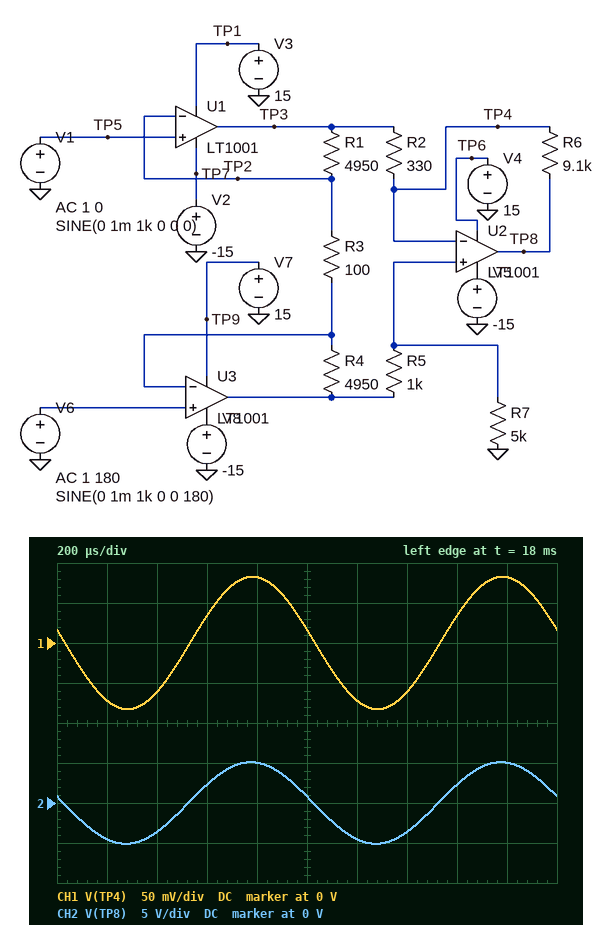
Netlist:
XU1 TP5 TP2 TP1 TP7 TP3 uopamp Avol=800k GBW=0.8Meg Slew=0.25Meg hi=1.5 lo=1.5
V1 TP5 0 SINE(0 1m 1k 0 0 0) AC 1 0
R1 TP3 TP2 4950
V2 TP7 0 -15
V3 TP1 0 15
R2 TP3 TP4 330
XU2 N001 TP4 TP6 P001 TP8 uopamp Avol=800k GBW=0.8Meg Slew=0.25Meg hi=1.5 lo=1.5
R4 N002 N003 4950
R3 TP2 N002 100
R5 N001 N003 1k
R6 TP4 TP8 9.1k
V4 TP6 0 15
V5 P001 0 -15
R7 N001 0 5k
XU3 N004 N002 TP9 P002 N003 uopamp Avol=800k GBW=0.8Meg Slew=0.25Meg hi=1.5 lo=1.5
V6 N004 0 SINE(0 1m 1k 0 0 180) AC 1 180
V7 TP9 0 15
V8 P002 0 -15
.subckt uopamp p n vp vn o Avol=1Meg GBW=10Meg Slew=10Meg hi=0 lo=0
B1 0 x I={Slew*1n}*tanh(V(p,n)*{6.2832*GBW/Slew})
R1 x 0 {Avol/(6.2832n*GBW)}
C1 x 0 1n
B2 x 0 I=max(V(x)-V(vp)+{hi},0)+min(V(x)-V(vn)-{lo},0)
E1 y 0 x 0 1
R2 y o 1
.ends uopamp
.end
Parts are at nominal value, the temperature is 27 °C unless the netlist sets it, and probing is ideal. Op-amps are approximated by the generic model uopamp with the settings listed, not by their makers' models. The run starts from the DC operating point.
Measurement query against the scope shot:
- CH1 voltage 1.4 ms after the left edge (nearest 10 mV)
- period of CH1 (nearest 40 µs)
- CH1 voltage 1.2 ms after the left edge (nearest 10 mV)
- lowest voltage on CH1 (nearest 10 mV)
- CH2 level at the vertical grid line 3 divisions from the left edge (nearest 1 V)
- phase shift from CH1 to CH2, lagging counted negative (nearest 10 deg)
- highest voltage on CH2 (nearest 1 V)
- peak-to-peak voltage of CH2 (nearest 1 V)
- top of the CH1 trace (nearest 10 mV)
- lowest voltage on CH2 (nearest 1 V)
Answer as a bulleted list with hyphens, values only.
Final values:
- -60 mV
- 1.00 ms
- -70 mV
- -80 mV
- 2 V
- 0 deg
- 5 V
- 10 V
- 80 mV
- -5 V
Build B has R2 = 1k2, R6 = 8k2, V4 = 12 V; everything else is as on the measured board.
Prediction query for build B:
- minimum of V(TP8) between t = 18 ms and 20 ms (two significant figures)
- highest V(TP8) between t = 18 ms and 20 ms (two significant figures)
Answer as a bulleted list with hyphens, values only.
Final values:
- -1.3 V
- 1.3 V
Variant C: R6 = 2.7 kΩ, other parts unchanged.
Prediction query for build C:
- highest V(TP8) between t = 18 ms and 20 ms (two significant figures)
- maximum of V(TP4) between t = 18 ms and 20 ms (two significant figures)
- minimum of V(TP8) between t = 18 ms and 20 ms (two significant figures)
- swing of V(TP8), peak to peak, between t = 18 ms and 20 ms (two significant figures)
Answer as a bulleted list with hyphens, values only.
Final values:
- 1.6 V
- 83 mV
- -1.6 V
- 3.1 V
